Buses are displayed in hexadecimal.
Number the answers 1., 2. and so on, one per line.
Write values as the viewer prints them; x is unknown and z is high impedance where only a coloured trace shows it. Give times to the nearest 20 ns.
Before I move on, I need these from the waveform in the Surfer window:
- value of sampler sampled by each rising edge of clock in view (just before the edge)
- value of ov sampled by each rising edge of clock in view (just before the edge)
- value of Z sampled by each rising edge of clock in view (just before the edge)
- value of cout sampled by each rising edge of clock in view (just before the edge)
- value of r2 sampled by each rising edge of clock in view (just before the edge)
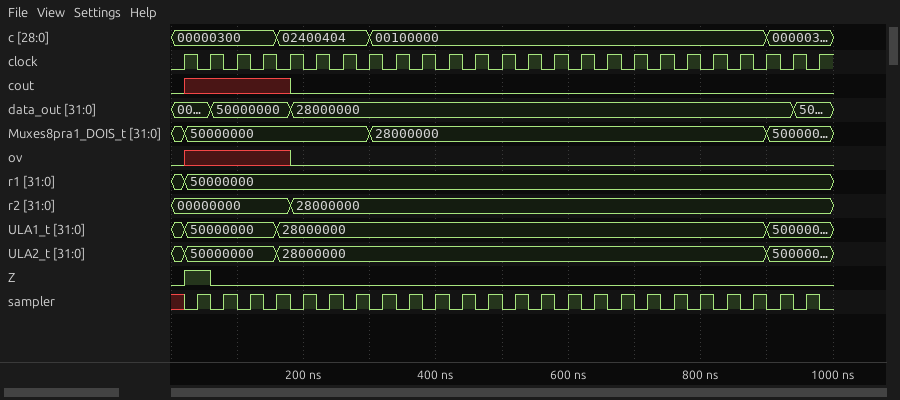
1. x 1 1 1 1 1 1 1 1 1 1 1 1 1 1 1 1 1 1 1 1 1 1 1 1
2. 0 x x x x 0 0 0 0 0 0 0 0 0 0 0 0 0 0 0 0 0 0 0 0
3. 0 1 0 0 0 0 0 0 0 0 0 0 0 0 0 0 0 0 0 0 0 0 0 0 0
4. 0 x x x x 0 0 0 0 0 0 0 0 0 0 0 0 0 0 0 0 0 0 0 0
5. 00000000, 00000000, 00000000, 00000000, 00000000, 28000000, 28000000, 28000000, 28000000, 28000000, 28000000, 28000000, 28000000, 28000000, 28000000, 28000000, 28000000, 28000000, 28000000, 28000000, 28000000, 28000000, 28000000, 28000000, 28000000
